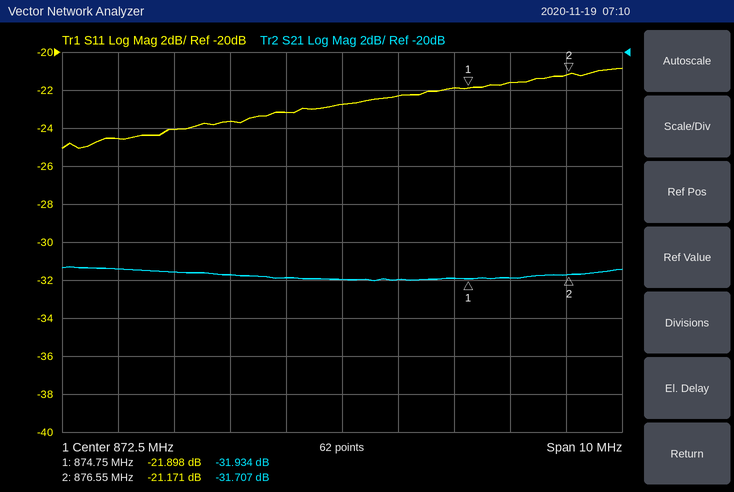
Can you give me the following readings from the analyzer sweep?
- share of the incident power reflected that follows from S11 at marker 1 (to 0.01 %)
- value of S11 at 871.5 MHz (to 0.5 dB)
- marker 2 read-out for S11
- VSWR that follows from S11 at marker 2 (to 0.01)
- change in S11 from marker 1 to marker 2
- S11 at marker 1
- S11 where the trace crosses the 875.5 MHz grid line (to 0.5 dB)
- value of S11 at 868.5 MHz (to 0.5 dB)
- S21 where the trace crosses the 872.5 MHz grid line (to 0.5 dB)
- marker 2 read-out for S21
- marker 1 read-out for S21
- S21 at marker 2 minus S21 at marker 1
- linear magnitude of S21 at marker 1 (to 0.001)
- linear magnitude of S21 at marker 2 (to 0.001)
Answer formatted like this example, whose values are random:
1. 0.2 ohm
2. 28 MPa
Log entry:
1. 0.65 %
2. -23.0 dB
3. -21.171 dB
4. 1.19
5. 0.727 dB
6. -21.898 dB
7. -21.5 dB
8. -24.5 dB
9. -32.0 dB
10. -31.707 dB
11. -31.934 dB
12. 0.227 dB
13. 0.025
14. 0.026
